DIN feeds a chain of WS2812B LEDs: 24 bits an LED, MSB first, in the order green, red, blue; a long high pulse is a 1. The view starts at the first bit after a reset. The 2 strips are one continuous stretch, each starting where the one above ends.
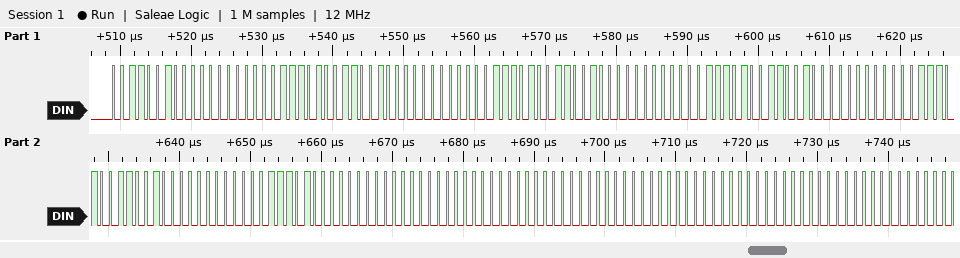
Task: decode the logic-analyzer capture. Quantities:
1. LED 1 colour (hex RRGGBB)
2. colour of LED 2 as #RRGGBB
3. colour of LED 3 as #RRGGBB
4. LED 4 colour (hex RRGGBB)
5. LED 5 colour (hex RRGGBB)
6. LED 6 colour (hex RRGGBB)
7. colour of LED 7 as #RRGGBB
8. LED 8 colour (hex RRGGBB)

#00321D
#00321D
#00321D
#00321D
#00321D
#000000
#000000
#000000
